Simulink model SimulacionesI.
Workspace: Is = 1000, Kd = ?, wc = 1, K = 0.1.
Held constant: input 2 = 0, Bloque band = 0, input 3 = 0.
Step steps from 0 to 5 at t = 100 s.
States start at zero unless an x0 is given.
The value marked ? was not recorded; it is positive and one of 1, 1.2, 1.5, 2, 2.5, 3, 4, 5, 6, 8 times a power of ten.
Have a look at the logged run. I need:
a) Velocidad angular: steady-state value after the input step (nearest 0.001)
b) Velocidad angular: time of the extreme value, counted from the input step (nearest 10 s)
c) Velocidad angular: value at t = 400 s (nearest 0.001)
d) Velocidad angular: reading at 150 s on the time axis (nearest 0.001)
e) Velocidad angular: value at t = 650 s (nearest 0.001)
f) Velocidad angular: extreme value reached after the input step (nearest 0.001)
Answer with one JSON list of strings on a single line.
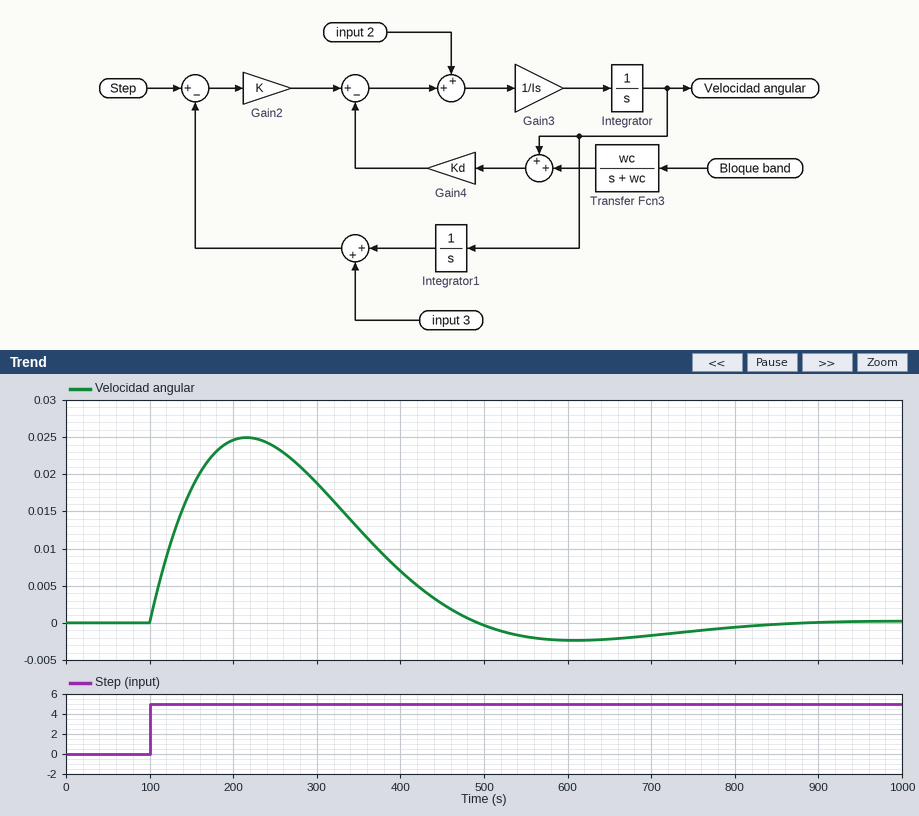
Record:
["0.000", "120 s", "0.007", "0.018", "-0.002", "0.025"]
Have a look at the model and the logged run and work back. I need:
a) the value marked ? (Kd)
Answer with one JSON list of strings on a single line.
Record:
["12"]
